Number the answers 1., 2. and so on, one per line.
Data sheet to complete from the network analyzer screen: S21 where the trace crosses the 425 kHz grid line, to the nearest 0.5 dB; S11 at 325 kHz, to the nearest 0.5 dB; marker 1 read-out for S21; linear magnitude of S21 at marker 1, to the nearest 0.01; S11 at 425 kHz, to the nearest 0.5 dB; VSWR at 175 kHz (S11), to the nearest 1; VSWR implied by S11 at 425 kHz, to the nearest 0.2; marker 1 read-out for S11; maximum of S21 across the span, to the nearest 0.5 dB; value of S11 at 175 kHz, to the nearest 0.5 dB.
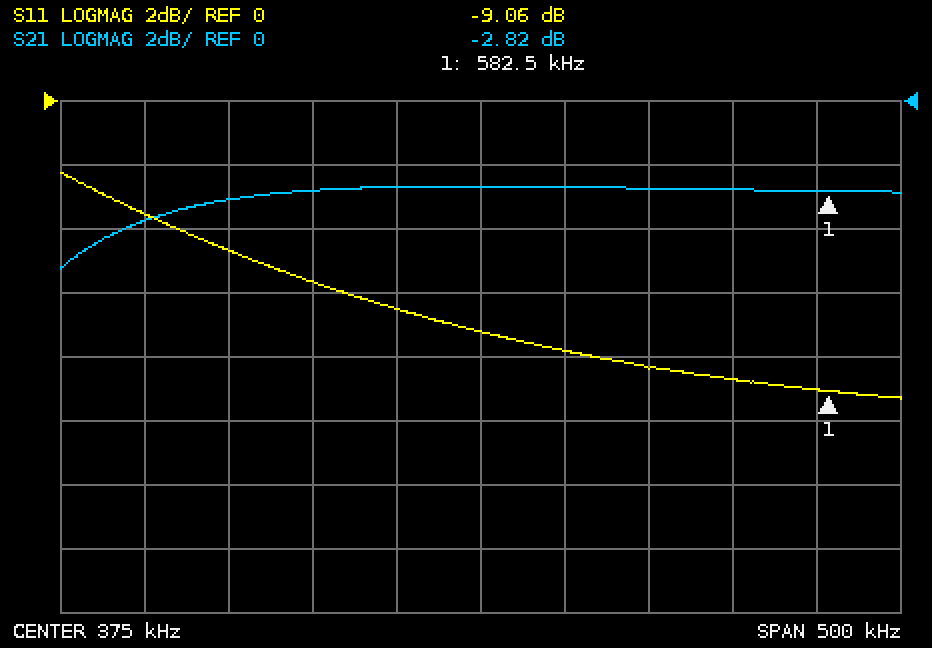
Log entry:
1. -2.5 dB
2. -6.5 dB
3. -2.82 dB
4. 0.72
5. -8.0 dB
6. 5
7. 2.4
8. -9.06 dB
9. -2.5 dB
10. -3.5 dB
